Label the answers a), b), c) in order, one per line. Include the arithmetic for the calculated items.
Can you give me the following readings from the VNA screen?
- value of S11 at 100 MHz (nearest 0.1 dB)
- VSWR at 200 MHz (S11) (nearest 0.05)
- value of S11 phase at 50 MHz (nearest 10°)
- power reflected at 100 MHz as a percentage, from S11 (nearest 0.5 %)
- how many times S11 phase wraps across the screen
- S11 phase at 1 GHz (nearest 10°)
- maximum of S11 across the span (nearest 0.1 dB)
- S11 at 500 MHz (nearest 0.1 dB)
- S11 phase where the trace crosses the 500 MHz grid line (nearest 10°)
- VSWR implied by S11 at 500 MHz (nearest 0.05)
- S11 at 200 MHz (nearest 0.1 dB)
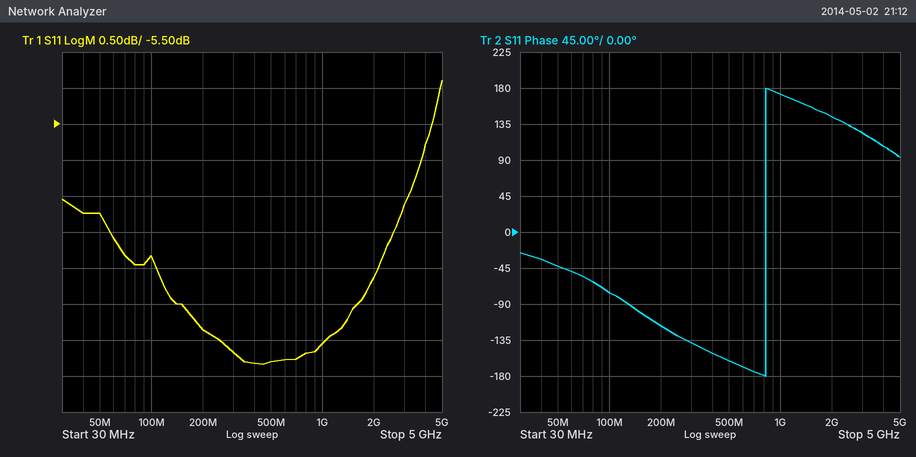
a) -7.3 dB
b) |Γ| = 10^(-8.4/20) = 0.3802; VSWR = (1 + 0.3802)/(1 − 0.3802) ≈ 2.23, so 2.25 to the nearest 0.05
c) -40°
d) 10^(-7.3/10) ≈ 18.6 %, so 18.5 % to the nearest 0.5 %
e) 1
f) 170°
g) -4.9 dB
h) -8.8 dB
i) -160°
j) |Γ| = 10^(-8.8/20) = 0.3631; VSWR = (1 + 0.3631)/(1 − 0.3631) ≈ 2.14, so 2.15 to the nearest 0.05
k) -8.4 dB
